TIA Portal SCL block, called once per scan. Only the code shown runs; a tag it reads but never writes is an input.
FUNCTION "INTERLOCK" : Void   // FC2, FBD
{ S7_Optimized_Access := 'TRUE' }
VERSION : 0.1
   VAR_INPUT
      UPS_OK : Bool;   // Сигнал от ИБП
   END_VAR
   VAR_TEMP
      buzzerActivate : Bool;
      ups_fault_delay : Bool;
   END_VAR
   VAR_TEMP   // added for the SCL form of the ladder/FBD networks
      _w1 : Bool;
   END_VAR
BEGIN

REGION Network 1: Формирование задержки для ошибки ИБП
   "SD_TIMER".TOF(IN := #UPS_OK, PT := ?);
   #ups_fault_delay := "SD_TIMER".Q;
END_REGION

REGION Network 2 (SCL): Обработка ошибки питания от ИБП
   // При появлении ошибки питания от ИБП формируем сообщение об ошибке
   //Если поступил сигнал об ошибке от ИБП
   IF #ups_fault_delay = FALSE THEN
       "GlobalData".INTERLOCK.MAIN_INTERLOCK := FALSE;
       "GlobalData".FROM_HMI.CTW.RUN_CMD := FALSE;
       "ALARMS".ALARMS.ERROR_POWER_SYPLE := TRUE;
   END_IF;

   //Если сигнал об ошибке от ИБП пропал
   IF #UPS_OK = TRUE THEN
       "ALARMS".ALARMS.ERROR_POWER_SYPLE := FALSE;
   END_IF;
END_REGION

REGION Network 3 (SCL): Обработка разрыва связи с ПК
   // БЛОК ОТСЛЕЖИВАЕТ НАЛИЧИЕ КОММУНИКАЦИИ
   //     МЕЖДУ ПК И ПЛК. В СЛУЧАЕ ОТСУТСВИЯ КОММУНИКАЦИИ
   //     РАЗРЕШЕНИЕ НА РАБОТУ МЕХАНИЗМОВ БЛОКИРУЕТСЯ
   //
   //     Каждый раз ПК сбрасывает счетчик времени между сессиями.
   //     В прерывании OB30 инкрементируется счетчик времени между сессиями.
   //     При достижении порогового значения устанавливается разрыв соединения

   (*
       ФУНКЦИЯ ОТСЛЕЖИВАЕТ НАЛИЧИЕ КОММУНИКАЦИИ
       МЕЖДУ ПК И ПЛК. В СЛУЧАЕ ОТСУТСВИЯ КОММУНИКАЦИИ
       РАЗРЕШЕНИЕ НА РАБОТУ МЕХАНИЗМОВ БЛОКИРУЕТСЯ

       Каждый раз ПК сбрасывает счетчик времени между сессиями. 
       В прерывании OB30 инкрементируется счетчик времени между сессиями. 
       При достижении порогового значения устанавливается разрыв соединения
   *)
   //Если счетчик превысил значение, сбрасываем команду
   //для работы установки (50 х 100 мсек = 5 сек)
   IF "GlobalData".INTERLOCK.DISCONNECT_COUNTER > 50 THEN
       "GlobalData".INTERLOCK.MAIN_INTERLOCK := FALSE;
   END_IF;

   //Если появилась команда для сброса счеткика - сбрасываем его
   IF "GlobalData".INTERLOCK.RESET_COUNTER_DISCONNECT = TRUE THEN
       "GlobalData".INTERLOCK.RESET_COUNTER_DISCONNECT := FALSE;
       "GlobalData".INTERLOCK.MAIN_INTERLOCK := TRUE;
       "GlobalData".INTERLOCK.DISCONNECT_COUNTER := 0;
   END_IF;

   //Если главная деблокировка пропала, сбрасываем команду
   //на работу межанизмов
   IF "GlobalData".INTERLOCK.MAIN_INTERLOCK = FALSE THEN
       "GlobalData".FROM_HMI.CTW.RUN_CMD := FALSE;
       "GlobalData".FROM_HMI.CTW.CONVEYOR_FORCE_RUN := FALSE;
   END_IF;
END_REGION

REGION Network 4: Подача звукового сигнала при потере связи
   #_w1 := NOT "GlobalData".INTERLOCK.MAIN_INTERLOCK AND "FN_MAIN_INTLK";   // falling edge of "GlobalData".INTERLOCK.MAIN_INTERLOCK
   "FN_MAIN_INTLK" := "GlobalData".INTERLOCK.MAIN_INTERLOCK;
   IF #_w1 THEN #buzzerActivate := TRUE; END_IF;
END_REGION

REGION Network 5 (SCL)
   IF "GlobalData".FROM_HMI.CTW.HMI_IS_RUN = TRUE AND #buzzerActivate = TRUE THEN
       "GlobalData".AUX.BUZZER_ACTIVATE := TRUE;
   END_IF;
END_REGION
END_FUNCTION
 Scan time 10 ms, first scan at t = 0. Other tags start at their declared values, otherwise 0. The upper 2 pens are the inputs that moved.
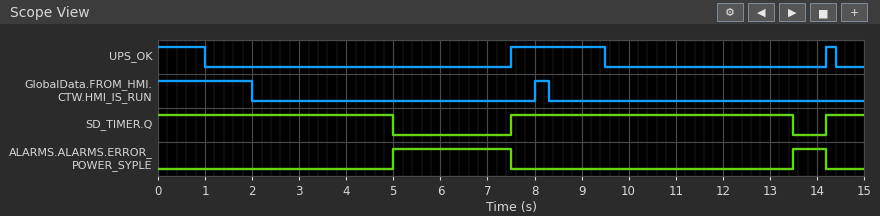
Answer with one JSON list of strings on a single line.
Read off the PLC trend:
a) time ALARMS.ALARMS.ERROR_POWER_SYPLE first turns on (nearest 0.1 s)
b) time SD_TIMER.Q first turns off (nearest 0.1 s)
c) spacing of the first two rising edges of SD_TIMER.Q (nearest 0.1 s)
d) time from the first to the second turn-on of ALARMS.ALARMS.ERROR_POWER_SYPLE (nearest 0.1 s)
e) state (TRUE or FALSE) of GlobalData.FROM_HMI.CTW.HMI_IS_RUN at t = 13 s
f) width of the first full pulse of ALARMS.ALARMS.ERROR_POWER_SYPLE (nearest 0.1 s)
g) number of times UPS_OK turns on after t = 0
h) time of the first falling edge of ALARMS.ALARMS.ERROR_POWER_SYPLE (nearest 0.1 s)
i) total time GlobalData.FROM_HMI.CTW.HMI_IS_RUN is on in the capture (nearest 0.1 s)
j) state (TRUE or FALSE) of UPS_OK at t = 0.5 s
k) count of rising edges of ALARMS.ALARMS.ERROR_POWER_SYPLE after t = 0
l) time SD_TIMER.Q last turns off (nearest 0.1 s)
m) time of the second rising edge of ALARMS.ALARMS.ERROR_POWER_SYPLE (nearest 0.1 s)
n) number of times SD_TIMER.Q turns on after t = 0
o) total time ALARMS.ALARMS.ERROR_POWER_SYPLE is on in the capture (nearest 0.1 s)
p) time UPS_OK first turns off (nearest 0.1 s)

["5.0 s", "5.0 s", "6.7 s", "8.5 s", "FALSE", "2.5 s", "2", "7.5 s", "2.3 s", "TRUE", "2", "13.5 s", "13.5 s", "2", "3.2 s", "1.0 s"]
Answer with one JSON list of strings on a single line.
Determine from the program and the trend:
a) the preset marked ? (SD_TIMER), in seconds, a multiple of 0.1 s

["4.0 s"]
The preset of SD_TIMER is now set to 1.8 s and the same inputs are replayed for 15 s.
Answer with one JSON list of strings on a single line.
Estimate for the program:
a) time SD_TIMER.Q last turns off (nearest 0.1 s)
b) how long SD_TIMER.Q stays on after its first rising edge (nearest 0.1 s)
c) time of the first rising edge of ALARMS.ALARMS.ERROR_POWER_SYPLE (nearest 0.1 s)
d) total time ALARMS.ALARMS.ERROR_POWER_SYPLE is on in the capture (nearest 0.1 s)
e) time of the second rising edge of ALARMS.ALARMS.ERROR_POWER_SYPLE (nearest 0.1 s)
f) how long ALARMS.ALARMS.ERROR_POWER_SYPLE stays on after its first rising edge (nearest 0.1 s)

["11.3 s", "3.8 s", "2.8 s", "7.6 s", "11.3 s", "4.7 s"]
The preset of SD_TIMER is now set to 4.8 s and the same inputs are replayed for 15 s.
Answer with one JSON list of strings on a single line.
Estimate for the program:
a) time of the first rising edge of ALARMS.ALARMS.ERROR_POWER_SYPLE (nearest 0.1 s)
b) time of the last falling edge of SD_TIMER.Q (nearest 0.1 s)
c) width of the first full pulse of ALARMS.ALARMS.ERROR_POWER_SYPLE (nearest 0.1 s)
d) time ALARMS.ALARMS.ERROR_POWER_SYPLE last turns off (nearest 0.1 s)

["5.8 s", "5.8 s", "1.7 s", "7.5 s"]
